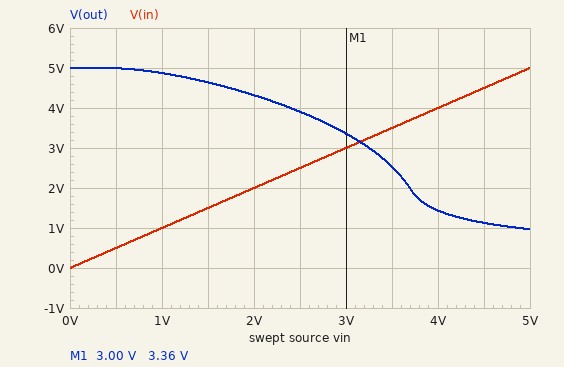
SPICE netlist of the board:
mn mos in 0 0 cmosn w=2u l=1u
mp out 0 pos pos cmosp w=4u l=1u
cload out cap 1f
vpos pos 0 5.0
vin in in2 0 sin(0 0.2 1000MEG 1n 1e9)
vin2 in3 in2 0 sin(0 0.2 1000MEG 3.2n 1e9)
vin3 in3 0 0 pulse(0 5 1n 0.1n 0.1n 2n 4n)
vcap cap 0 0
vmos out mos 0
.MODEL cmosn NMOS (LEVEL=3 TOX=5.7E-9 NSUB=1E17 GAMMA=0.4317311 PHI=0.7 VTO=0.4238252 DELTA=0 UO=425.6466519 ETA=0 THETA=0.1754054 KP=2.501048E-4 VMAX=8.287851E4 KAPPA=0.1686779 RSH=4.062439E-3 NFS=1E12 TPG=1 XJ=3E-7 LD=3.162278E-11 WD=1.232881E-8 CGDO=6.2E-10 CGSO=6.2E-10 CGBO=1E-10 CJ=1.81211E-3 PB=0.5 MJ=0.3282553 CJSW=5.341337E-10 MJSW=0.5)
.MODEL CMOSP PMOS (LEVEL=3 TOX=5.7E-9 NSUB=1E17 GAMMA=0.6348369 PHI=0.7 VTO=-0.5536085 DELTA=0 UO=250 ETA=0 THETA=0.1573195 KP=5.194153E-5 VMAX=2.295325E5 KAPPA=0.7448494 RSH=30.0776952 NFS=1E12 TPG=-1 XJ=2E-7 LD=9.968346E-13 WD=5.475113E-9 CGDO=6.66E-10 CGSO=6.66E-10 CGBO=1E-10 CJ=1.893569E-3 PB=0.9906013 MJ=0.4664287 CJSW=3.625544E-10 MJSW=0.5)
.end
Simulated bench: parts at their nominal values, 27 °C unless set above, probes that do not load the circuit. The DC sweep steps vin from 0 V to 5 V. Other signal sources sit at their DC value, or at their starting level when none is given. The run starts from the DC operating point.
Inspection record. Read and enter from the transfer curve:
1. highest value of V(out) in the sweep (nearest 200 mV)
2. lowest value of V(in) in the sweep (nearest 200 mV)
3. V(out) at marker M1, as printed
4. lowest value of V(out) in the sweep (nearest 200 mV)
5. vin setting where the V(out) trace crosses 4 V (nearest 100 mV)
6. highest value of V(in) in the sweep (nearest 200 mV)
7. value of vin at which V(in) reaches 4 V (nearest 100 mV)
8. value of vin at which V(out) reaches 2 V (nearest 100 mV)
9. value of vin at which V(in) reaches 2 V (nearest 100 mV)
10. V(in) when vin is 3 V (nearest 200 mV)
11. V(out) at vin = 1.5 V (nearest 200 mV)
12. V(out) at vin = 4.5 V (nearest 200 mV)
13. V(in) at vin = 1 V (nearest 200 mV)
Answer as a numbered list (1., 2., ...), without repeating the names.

1. 5.0 V
2. 0 V
3. 3.36 V
4. 1.0 V
5. 2.4 V
6. 5.0 V
7. 4.0 V
8. 3.7 V
9. 2.0 V
10. 3.0 V
11. 4.6 V
12. 1.2 V
13. 1.0 V
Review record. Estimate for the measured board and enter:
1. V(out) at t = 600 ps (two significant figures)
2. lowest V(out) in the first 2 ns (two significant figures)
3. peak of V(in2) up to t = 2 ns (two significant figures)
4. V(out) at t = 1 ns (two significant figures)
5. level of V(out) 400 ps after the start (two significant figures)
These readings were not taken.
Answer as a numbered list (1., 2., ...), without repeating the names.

1. 5.0 V
2. 930 mV
3. 5.0 V
4. 5.0 V
5. 5.0 V
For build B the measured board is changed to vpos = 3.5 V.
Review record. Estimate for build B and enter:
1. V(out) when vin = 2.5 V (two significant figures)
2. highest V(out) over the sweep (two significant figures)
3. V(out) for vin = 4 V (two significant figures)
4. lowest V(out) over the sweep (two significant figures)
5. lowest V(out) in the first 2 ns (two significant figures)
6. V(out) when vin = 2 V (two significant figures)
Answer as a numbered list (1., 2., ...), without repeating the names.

1. 1.5 V
2. 3.5 V
3. 530 mV
4. 430 mV
5. 410 mV
6. 2.5 V
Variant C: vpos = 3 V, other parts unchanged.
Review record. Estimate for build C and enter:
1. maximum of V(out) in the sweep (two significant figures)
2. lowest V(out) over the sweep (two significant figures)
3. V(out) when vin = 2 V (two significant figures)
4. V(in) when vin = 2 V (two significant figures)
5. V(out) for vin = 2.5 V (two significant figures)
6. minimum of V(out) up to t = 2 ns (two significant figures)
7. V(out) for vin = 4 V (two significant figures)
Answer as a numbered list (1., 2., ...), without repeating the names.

1. 3.0 V
2. 300 mV
3. 1.7 V
4. 2.0 V
5. 680 mV
6. 290 mV
7. 370 mV
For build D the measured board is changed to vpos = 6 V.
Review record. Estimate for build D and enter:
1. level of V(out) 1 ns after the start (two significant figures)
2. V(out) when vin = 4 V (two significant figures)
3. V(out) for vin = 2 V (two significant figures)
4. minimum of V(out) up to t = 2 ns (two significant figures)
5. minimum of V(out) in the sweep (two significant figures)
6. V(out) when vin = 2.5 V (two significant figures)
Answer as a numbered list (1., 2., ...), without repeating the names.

1. 6.0 V
2. 3.5 V
3. 5.4 V
4. 1.5 V
5. 1.6 V
6. 5.1 V
